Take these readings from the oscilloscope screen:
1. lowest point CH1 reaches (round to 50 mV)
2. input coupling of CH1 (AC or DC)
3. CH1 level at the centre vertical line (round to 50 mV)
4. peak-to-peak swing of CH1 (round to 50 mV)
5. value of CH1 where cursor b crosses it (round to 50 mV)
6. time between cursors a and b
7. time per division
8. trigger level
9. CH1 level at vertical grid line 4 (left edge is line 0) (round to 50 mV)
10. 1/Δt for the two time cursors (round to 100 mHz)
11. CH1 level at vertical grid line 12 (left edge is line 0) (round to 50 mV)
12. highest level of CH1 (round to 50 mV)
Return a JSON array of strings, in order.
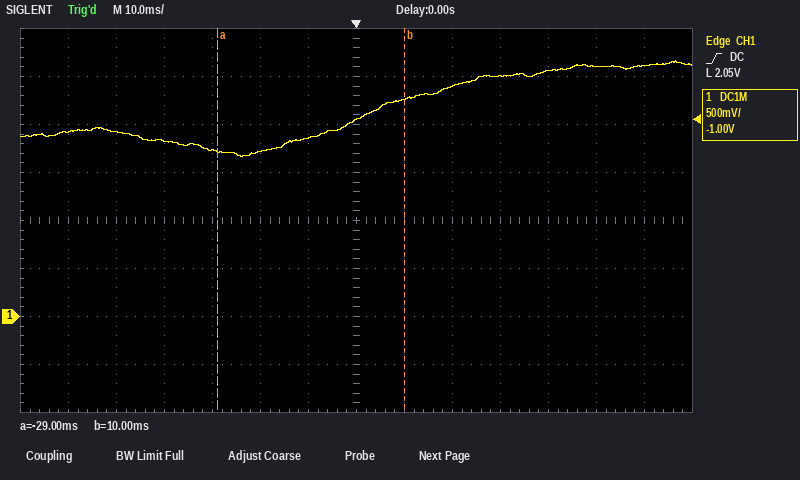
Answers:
["1.65 V", "DC", "2.05 V", "1.00 V", "2.25 V", "39 ms", "10 ms", "2.05 V", "1.75 V", "25.6 Hz", "2.60 V", "2.65 V"]
